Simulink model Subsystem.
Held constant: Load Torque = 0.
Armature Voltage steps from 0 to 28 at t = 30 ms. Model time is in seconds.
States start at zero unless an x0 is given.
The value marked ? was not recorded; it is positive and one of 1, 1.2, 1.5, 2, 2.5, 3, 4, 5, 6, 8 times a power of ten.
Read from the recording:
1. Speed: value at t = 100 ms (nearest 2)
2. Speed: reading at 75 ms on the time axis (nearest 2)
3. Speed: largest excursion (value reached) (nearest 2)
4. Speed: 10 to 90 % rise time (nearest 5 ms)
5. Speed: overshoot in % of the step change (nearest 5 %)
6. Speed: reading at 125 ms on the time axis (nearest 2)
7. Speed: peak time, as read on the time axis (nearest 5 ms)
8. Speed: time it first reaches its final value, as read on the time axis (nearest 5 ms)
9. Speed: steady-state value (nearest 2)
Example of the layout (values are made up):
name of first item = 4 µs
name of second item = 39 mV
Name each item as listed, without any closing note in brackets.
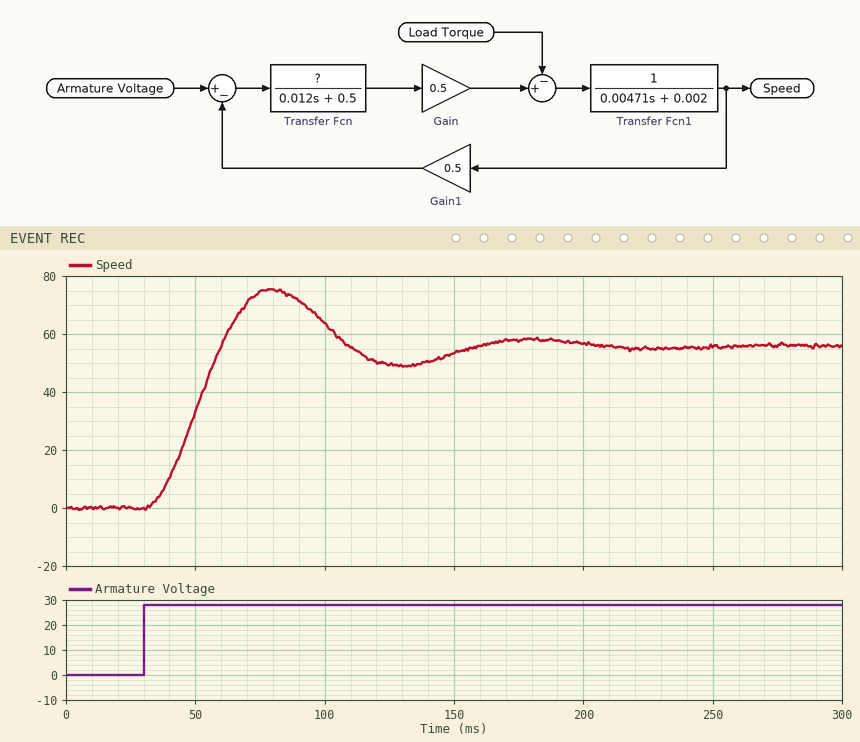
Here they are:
Speed: value at t = 100 ms = 64
Speed: reading at 75 ms on the time axis = 74
Speed: largest excursion (value reached) = 76
Speed: 10 to 90 % rise time = 20 ms
Speed: overshoot in % of the step change = 35 %
Speed: reading at 125 ms on the time axis = 50
Speed: peak time, as read on the time axis = 80 ms
Speed: time it first reaches its final value, as read on the time axis = 60 ms
Speed: steady-state value = 56
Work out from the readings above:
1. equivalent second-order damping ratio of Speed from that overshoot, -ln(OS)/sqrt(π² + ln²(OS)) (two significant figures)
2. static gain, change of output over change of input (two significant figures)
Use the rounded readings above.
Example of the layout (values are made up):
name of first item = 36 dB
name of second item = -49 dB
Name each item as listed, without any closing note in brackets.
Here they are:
equivalent second-order damping ratio of Speed from that overshoot, -ln(OS)/sqrt(π² + ln²(OS)) = 0.32
static gain, change of output over change of input = 2.0
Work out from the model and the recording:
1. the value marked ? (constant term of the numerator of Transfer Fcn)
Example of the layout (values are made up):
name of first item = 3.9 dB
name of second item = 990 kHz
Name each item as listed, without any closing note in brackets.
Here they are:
the value marked ? = 1
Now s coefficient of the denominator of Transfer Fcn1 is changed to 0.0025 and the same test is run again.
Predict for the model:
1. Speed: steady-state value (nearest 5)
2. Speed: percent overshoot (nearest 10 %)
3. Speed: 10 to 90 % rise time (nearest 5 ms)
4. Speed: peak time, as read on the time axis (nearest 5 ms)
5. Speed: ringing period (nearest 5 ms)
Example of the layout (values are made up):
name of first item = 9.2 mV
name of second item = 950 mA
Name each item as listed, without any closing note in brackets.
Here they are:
Speed: steady-state value = 55
Speed: percent overshoot = 50 %
Speed: 10 to 90 % rise time = 15 ms
Speed: peak time, as read on the time axis = 65 ms
Speed: ringing period = 70 ms
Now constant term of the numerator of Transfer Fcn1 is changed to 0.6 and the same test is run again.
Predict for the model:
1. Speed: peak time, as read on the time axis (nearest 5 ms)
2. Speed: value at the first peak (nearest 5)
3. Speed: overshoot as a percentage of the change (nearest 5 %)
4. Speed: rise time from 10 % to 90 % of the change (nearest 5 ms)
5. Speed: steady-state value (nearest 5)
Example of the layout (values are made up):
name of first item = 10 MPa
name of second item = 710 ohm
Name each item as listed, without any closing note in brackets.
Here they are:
Speed: peak time, as read on the time axis = 95 ms
Speed: value at the first peak = 70
Speed: overshoot as a percentage of the change = 25 %
Speed: rise time from 10 % to 90 % of the change = 30 ms
Speed: steady-state value = 55
